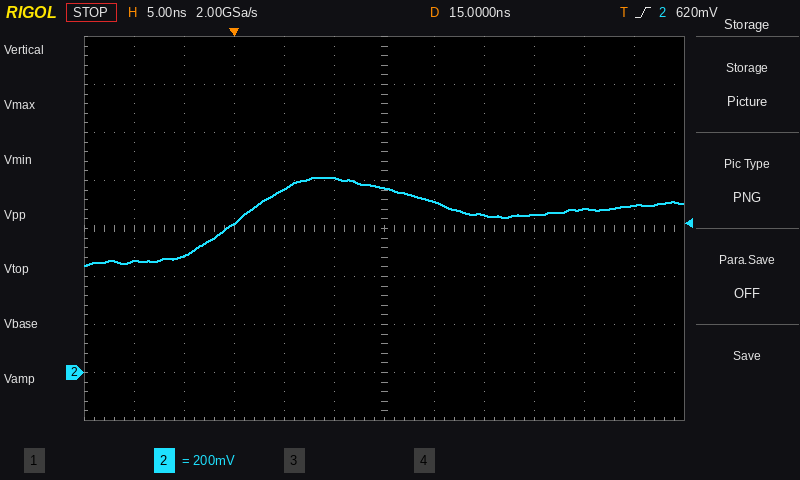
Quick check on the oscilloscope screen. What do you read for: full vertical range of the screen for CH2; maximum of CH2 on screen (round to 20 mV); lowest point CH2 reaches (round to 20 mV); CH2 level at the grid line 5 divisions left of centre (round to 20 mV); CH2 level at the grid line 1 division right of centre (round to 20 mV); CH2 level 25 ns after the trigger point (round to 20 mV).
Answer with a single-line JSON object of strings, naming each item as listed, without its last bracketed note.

{"full vertical range of the screen for CH2": "1.6 V", "maximum of CH2 on screen": "820 mV", "lowest point CH2 reaches": "440 mV", "CH2 level at the grid line 5 divisions left of centre": "460 mV", "CH2 level at the grid line 1 division right of centre": "720 mV", "CH2 level 25 ns after the trigger point": "660 mV"}
